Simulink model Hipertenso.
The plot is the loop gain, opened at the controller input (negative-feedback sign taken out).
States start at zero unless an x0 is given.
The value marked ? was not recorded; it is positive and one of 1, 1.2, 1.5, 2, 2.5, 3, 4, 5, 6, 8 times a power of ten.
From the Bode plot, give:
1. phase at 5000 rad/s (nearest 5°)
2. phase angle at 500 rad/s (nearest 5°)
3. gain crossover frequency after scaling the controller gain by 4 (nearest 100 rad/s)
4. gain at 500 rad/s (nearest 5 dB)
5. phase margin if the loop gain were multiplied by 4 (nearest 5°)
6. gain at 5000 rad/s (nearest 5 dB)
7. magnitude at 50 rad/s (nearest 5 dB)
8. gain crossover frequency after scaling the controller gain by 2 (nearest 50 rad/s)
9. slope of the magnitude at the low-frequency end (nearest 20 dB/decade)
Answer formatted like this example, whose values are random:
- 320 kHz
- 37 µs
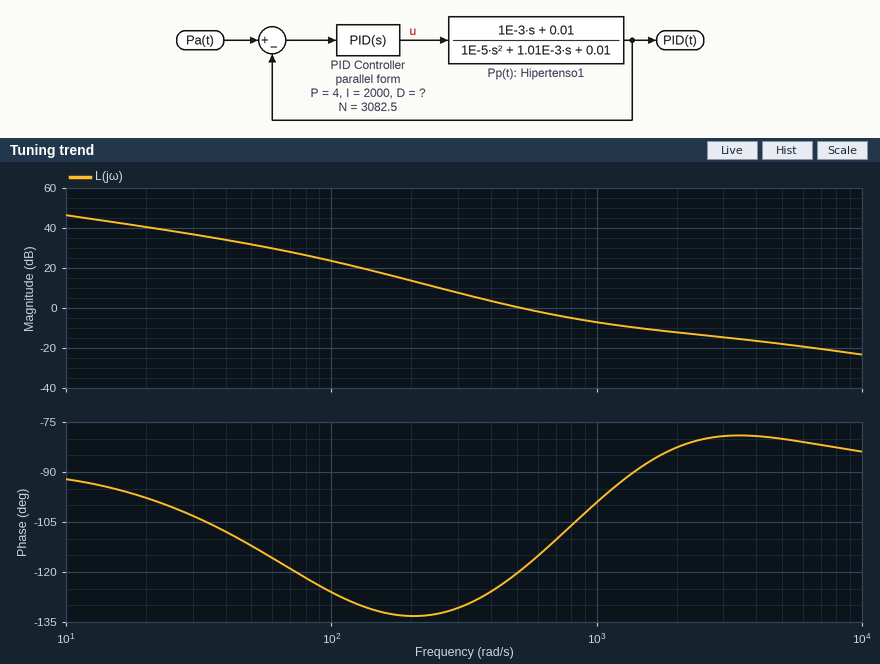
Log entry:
- -80°
- -120°
- 2000 rad/s
- 0 dB
- 95°
- -20 dB
- 30 dB
- 900 rad/s
- -20 dB/decade
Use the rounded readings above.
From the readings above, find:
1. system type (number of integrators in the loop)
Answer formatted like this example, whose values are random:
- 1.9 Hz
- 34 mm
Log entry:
- 1
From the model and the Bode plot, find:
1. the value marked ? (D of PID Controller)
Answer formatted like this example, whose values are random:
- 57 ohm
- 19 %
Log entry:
- 0.001
